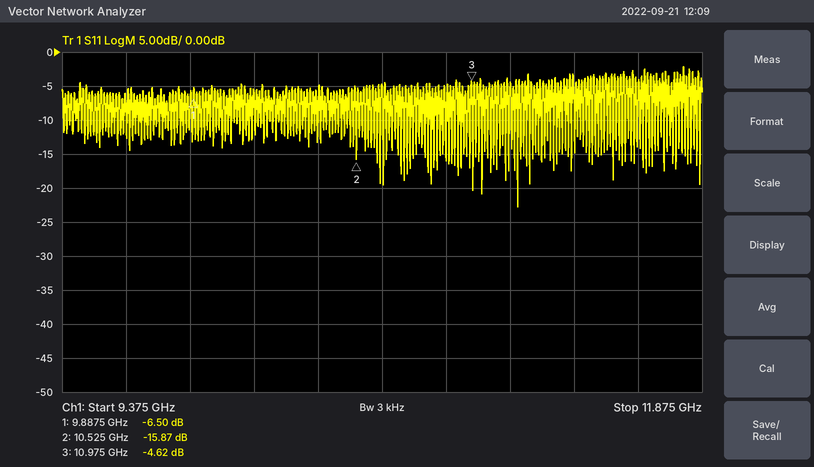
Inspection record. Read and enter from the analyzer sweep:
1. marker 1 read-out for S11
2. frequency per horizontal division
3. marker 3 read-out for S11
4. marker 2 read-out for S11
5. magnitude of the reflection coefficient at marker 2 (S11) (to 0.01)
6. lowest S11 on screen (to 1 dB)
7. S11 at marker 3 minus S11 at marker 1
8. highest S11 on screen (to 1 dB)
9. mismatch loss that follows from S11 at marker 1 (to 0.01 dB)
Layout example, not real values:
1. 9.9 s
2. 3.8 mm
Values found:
1. -6.50 dB
2. 250 MHz
3. -4.62 dB
4. -15.87 dB
5. 0.16
6. -23 dB
7. 1.88 dB
8. -2 dB
9. 1.10 dB
